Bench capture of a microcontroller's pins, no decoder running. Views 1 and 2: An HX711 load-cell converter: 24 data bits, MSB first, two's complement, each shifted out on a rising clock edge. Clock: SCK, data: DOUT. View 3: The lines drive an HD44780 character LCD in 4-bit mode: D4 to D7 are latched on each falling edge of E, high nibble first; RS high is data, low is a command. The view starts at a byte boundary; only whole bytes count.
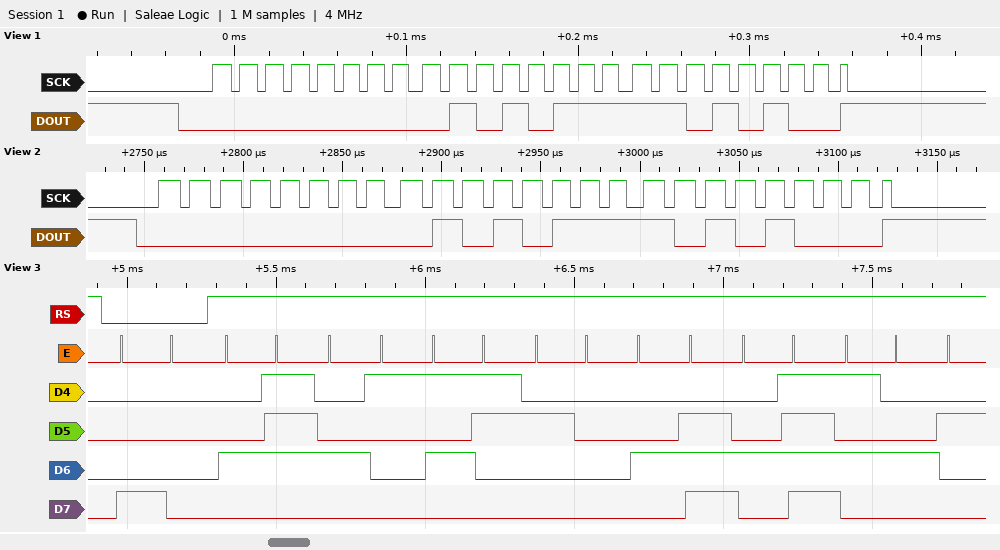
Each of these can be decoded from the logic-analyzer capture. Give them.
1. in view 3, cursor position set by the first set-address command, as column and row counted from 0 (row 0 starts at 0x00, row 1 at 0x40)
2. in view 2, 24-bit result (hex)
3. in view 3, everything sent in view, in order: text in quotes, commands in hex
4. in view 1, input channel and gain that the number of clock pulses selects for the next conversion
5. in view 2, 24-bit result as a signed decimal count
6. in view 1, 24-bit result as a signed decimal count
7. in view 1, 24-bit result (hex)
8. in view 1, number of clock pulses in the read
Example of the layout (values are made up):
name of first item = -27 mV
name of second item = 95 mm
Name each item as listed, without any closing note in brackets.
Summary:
in view 3, cursor position set by the first set-address command, as column and row counted from 0 = column 0, row 0
in view 2, 24-bit result = 0x0057A8
in view 3, everything sent in view, in order: text in quotes, commands in hex = 0x80 "GAS NOT"
in view 1, input channel and gain that the number of clock pulses selects for the next conversion = channel A, gain 128
in view 2, 24-bit result as a signed decimal count = 22440
in view 1, 24-bit result as a signed decimal count = 22484
in view 1, 24-bit result = 0x0057D4
in view 1, number of clock pulses in the read = 25
